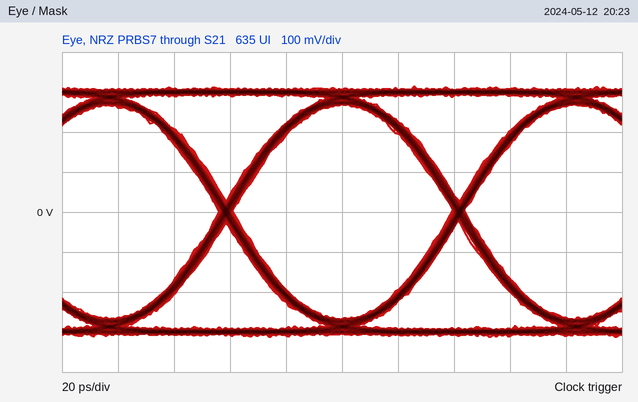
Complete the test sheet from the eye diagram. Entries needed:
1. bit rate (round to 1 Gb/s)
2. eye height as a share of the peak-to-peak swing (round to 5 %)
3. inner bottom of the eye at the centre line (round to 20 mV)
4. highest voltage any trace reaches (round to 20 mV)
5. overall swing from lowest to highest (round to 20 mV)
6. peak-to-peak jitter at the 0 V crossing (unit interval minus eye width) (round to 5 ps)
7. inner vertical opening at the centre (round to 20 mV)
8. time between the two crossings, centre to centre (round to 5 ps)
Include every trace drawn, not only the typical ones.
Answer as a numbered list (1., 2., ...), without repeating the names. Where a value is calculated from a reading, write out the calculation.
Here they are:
1. 12 Gb/s
2. 540 mV / 620 mV ≈ 87.1 %, so 85 % to the nearest 5 %
3. -260 mV
4. 320 mV
5. 620 mV
6. 5 ps
7. 540 mV
8. 85 ps
